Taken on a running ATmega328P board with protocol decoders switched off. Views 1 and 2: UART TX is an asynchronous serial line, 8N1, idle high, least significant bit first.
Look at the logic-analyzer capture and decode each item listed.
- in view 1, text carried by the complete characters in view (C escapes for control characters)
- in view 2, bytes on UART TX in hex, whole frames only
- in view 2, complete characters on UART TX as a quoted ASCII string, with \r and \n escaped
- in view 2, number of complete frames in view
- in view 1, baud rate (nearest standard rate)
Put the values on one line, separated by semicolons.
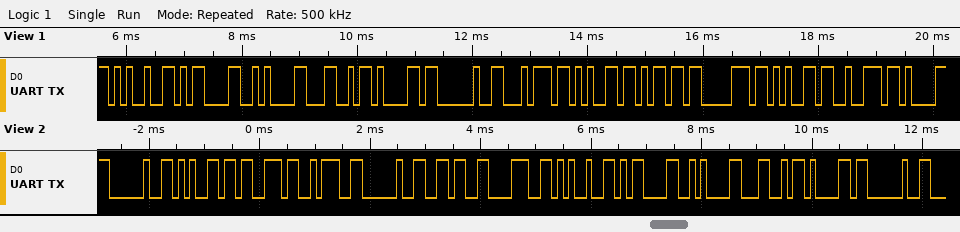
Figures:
"%\r\nLa temper"; 20 65 73 3A 20 36 38 25 0D 0A 4C 61 20; " es: 68%\r\nLa "; 13; 9600 baud
